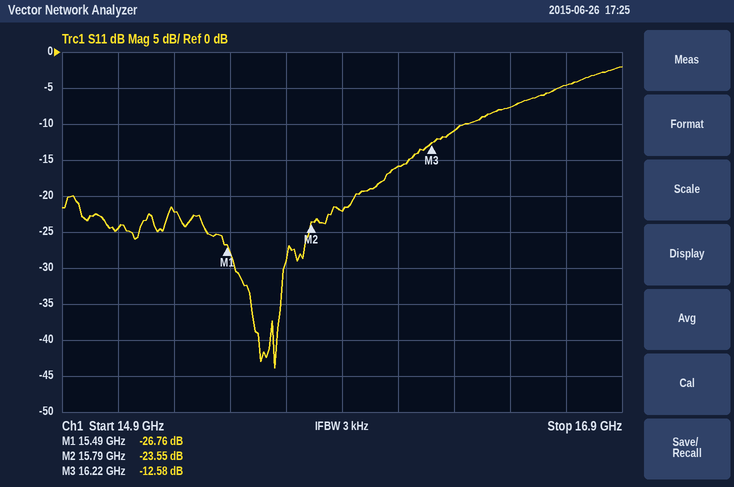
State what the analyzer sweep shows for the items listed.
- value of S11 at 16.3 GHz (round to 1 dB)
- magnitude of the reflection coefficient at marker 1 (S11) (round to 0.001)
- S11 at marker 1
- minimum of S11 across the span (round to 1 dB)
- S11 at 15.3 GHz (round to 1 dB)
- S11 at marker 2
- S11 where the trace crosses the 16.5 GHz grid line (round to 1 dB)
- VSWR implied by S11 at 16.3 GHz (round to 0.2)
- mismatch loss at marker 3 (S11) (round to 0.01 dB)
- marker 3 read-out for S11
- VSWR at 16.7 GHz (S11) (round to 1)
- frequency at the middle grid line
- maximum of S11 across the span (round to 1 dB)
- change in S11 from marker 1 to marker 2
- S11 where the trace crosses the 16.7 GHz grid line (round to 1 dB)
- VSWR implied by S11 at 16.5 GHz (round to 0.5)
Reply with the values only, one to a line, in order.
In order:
-11 dB
0.046
-26.76 dB
-44 dB
-22 dB
-23.55 dB
-8 dB
1.8
0.25 dB
-12.58 dB
4
15.9 GHz
-2 dB
3.21 dB
-5 dB
2.5
